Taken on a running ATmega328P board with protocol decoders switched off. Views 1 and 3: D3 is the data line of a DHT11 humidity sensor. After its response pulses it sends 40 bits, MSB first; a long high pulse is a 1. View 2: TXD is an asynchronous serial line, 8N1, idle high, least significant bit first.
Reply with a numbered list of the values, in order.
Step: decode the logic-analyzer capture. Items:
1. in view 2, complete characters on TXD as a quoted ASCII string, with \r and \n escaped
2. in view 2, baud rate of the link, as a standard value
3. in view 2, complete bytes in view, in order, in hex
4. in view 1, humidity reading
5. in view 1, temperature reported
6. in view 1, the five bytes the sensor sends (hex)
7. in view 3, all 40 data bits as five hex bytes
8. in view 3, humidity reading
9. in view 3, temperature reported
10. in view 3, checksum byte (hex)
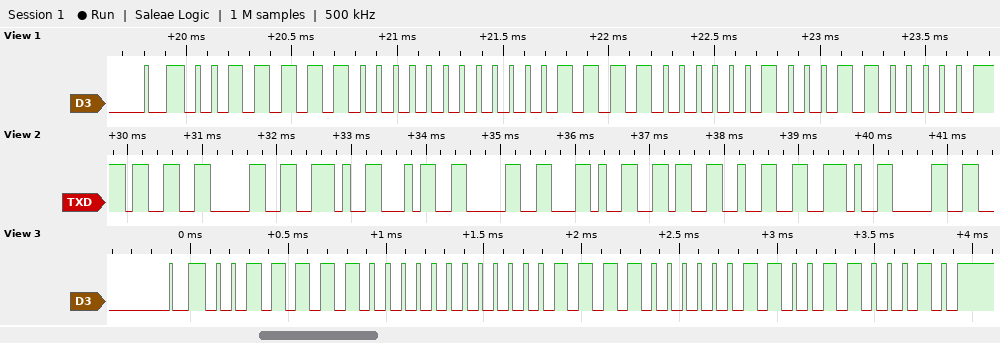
1. "30.40,62.0"
2. 9600 baud
3. 33 30 2E 34 30 2C 36 32 2E 30
4. 62 %
5. 30.4 °C
6. 3E 00 1E 04 60
7. 3E 00 1E 06 62
8. 62 %
9. 30.6 °C
10. 0x62
